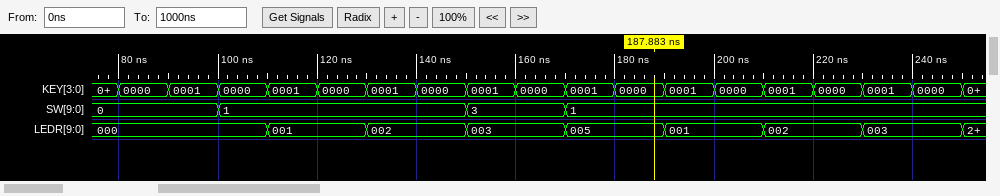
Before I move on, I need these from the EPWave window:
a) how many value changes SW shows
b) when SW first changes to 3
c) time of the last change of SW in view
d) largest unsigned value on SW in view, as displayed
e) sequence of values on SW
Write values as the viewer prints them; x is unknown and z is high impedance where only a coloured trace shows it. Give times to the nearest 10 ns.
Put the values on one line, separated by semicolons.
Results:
3; 150 ns; 170 ns; 3; 0, 1, 3, 1
